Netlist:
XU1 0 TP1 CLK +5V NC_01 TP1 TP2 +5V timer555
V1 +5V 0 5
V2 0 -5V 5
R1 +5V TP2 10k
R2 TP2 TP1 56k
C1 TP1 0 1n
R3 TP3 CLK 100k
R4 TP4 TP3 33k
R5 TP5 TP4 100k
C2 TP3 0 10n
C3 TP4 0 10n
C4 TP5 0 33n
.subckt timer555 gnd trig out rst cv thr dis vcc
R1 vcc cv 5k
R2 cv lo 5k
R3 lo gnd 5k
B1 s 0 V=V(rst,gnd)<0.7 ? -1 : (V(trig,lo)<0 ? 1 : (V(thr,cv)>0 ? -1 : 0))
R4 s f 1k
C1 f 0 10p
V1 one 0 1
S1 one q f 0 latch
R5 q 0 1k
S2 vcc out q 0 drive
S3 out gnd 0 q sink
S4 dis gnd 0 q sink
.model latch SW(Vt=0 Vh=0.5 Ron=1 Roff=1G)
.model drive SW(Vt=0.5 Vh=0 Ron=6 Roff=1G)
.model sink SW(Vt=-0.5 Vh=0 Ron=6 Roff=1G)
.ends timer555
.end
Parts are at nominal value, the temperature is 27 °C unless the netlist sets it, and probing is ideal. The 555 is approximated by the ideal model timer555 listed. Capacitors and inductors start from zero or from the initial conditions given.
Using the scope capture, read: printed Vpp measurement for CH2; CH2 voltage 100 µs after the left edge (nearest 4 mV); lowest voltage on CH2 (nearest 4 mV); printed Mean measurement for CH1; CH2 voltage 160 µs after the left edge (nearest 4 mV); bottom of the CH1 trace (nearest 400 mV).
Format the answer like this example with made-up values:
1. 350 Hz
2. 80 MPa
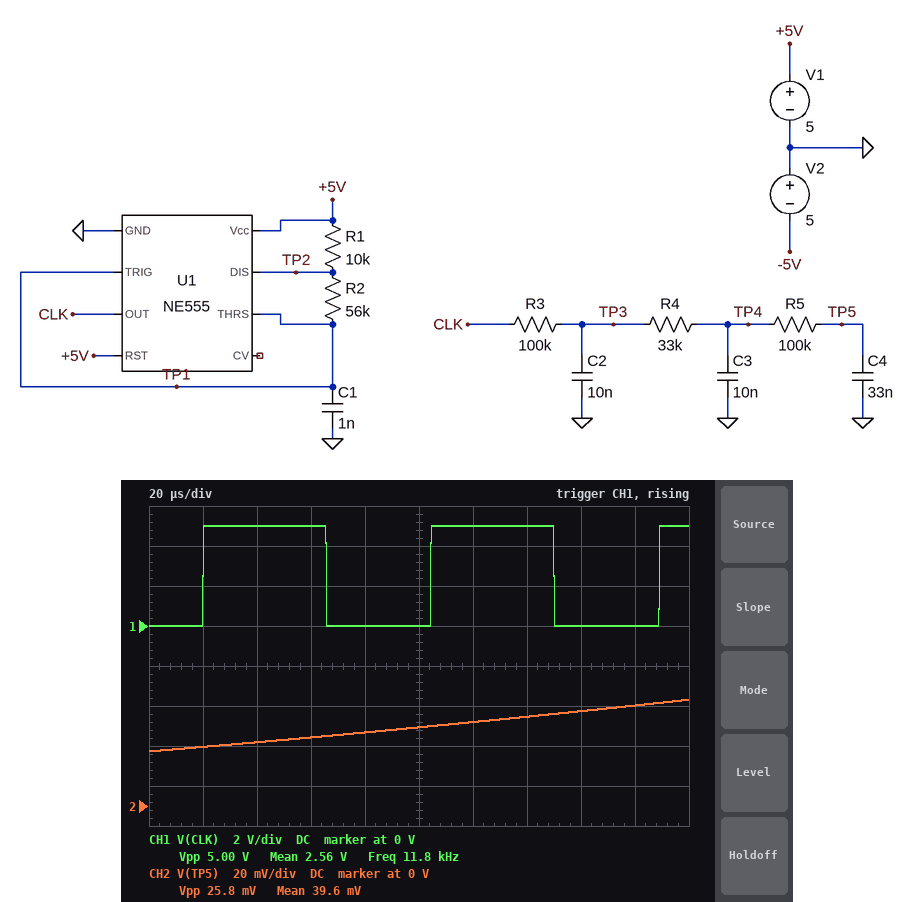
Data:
1. 25.8 mV
2. 40 mV
3. 28 mV
4. 2.56 V
5. 48 mV
6. 0 V
